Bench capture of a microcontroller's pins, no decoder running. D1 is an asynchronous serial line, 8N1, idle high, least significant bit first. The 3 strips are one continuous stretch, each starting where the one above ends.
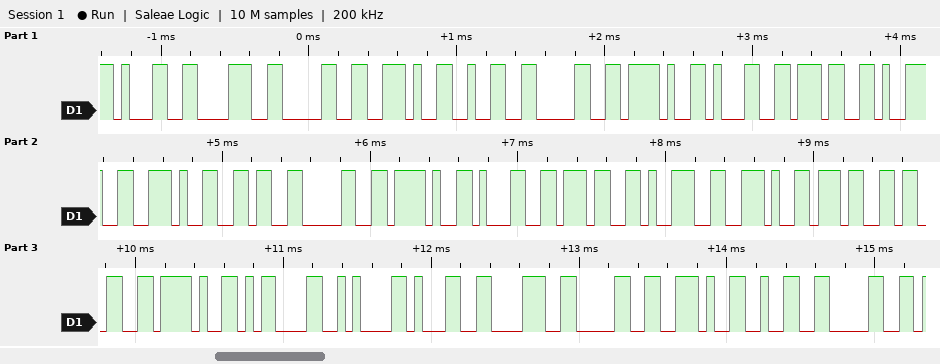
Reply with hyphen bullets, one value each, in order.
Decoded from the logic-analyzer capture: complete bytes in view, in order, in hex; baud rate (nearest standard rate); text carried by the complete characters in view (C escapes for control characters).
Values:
- 31 38 30 2E 32 30 2F 31 37 39 2E 36 30 2F 31 37 39 2E 37 33 2F 0D 0A 31 38 30 2E 32 30
- 19200 baud
- "180.20/179.60/179.73/\r\n180.20"
